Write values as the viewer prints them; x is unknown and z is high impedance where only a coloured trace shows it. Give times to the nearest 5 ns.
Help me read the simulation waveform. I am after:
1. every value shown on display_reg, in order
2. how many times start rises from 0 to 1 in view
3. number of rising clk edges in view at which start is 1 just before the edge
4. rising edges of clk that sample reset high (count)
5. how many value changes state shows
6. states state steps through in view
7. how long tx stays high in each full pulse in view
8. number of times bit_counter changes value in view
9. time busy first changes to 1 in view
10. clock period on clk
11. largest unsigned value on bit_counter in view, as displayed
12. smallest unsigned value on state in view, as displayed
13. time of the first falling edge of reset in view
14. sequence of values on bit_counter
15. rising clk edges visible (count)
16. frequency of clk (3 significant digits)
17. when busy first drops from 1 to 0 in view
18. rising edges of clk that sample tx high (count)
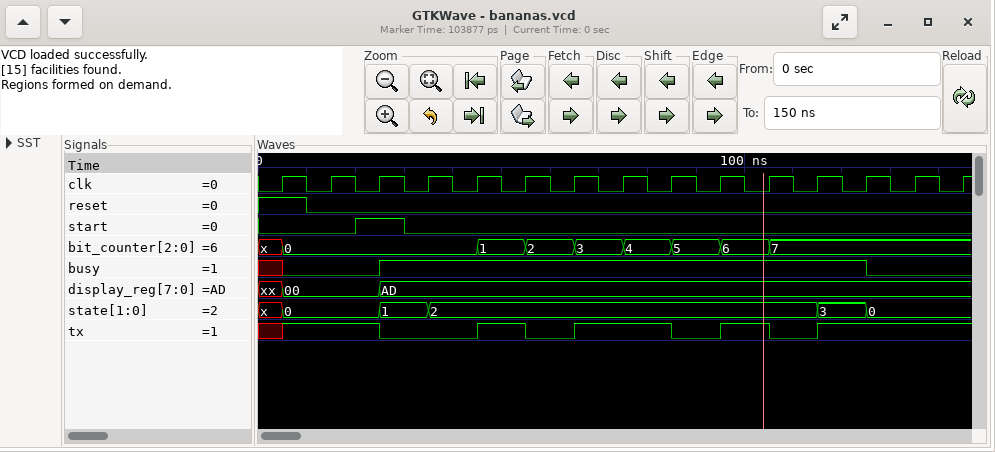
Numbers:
xx, 00, AD
1
1
1
5
x, 0, 1, 2, 3, 0
10 ns, 20 ns, 10 ns
8
25 ns
10 ns
7
0
10 ns
x, 0, 1, 2, 3, 4, 5, 6, 7
15
100 MHz
125 ns
9
